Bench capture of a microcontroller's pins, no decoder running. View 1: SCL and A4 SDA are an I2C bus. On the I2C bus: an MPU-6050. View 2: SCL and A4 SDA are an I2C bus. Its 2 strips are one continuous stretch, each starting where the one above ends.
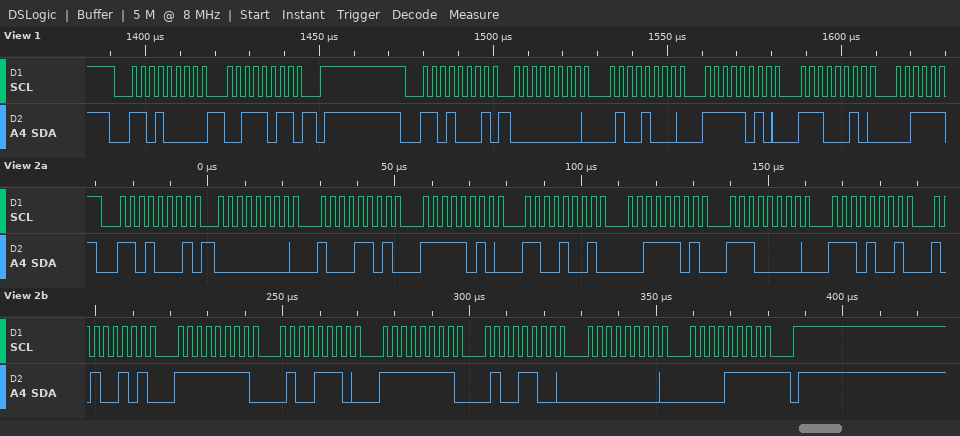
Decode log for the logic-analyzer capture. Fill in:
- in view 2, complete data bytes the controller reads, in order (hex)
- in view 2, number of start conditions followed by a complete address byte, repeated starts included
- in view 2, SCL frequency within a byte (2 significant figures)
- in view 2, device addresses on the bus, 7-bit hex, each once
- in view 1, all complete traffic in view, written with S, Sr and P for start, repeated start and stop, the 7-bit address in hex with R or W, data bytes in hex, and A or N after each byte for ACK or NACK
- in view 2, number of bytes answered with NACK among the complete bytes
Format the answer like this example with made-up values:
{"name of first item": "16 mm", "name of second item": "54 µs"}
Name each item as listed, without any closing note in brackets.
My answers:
{"in view 2, complete data bytes the controller reads, in order": "00 8D FA C9 3D E0 E9 A5 FF 4E FF 4C 00 0F", "in view 2, number of start conditions followed by a complete address byte, repeated starts included": "1", "in view 2, SCL frequency within a byte": "400 kHz", "in view 2, device addresses on the bus, 7-bit hex, each once": "0x68", "in view 1, all complete traffic in view, written with S, Sr and P for start, repeated start and stop, the 7-bit address in hex with R or W, data bytes in hex, and A or N after each byte for ACK or NACK": "S 68W A 3B A P S 68R A 00 A 48 A FA A E2 A", "in view 2, number of bytes answered with NACK among the complete bytes": "1"}
